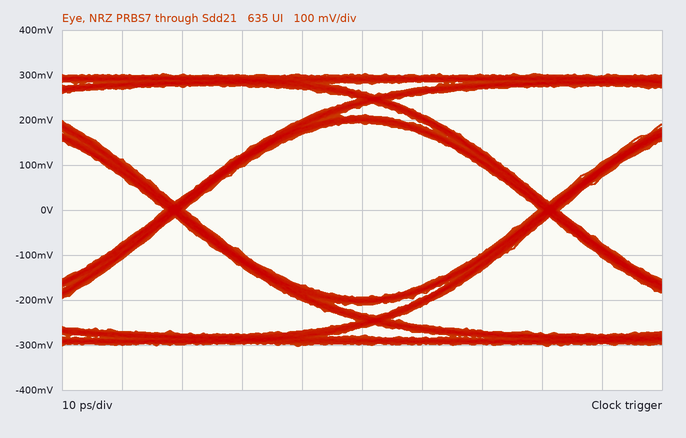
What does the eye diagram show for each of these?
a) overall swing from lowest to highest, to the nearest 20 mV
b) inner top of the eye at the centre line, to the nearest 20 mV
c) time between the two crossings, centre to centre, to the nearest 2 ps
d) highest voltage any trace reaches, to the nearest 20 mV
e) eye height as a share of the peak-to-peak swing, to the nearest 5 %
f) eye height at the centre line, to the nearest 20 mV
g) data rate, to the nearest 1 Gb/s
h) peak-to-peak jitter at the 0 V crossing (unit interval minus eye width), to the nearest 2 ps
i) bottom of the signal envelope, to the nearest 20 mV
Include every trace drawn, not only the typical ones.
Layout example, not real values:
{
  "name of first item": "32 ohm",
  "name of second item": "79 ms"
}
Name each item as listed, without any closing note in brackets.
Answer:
{
  "overall swing from lowest to highest, to the nearest 20 mV": "600 mV",
  "inner top of the eye at the centre line, to the nearest 20 mV": "200 mV",
  "time between the two crossings, centre to centre, to the nearest 2 ps": "62 ps",
  "highest voltage any trace reaches, to the nearest 20 mV": "300 mV",
  "eye height as a share of the peak-to-peak swing, to the nearest 5 %": "65 %",
  "eye height at the centre line, to the nearest 20 mV": "380 mV",
  "data rate, to the nearest 1 Gb/s": "16 Gb/s",
  "peak-to-peak jitter at the 0 V crossing (unit interval minus eye width), to the nearest 2 ps": "4 ps",
  "bottom of the signal envelope, to the nearest 20 mV": "-300 mV"
}
